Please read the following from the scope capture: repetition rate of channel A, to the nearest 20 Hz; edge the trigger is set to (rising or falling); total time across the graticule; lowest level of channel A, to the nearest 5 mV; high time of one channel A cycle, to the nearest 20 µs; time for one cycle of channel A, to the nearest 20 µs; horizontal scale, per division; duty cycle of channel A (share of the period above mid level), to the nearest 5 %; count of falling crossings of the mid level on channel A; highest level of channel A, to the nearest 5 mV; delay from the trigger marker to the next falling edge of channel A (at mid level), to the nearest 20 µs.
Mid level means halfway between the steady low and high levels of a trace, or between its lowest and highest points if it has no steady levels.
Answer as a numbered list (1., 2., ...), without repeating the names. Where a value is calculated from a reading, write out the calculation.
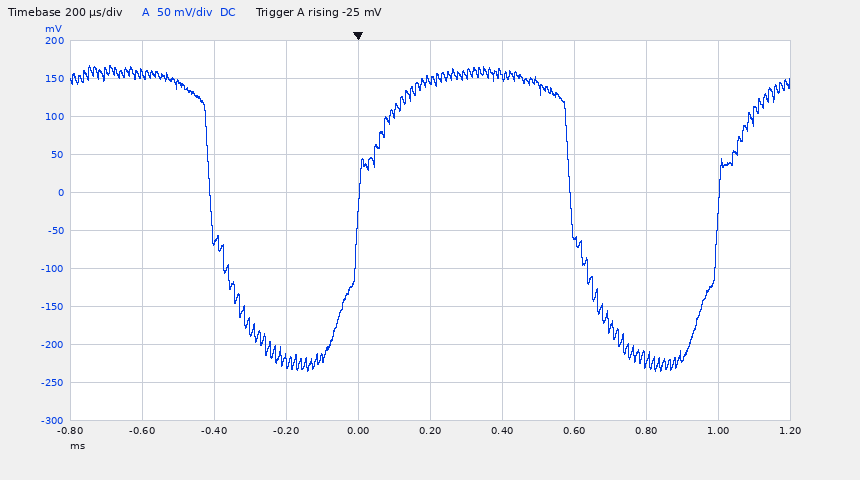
1. 1 / 1.00 ms ≈ 1.00 kHz
2. rising
3. 2 ms
4. -235 mV
5. 600 µs
6. 1.00 ms
7. 200 µs
8. 600 µs / 1.00 ms ≈ 60 %
9. 2
10. 165 mV
11. 600 µs
